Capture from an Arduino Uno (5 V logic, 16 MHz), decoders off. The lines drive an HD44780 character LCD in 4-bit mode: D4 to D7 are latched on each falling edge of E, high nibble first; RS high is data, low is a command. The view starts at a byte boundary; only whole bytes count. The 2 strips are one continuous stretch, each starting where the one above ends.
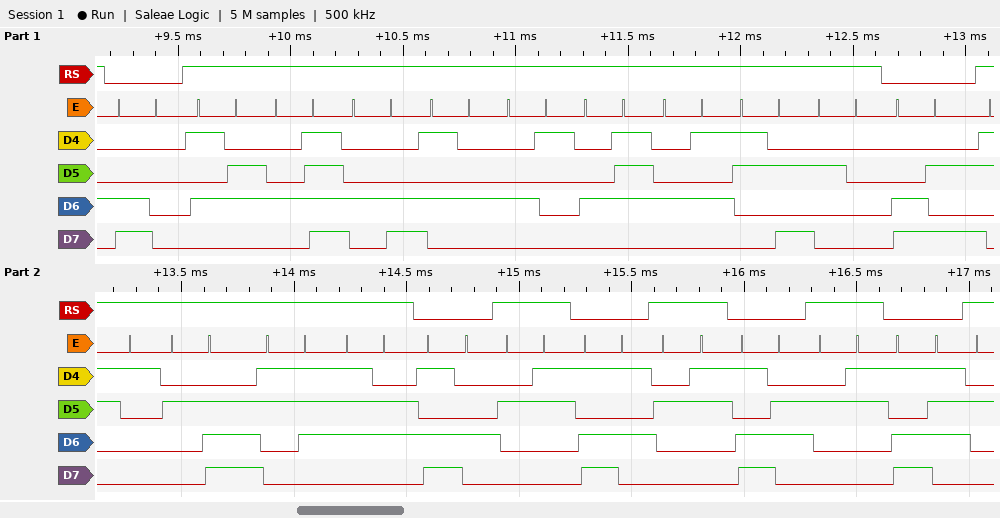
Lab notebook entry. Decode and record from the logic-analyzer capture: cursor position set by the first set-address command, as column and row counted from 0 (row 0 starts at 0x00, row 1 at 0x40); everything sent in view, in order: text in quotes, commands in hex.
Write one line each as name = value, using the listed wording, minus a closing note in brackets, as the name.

cursor position set by the first set-address command, as column and row counted from 0 = column 0, row 1
everything sent in view, in order: text in quotes, commands in hex = 0xC0 "VOLTAGE: " 0xCA "1.7v" 0xD4 "#" 0xD5 "#" 0xD6 "#" 0xD7
